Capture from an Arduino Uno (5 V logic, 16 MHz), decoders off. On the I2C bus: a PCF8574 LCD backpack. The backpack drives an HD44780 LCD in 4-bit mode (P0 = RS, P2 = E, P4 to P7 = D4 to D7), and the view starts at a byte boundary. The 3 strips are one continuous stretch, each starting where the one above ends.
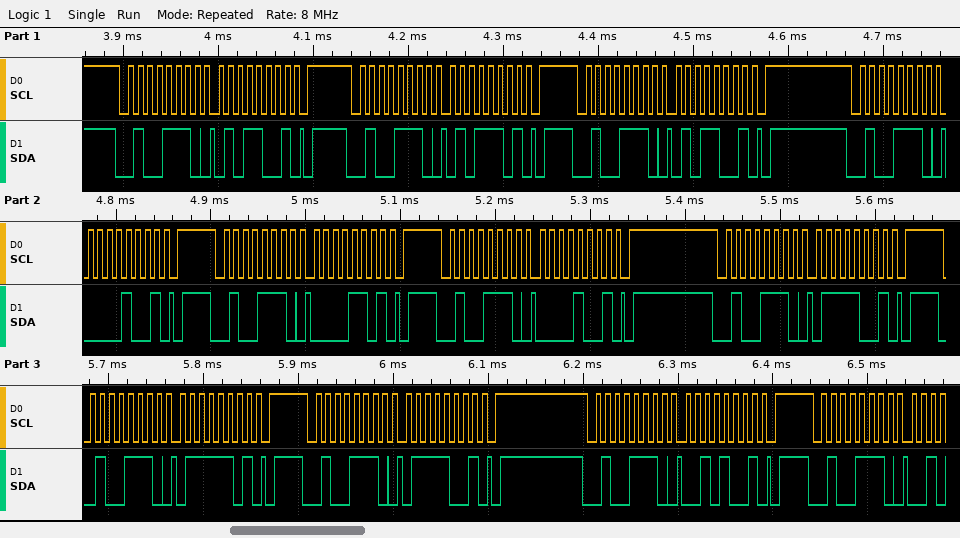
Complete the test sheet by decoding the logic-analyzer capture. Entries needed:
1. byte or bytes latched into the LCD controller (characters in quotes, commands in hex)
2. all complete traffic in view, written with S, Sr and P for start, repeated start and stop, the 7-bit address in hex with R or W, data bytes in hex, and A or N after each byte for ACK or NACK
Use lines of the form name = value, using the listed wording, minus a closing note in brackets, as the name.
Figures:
byte or bytes latched into the LCD controller = 'P'
all complete traffic in view, written with S, Sr and P for start, repeated start and stop, the 7-bit address in hex with R or W, data bytes in hex, and A or N after each byte for ACK or NACK = S 27W A 59 A P S 27W A 5D A P S 27W A 59 A P S 27W A 09 A P S 27W A 0D A P S 27W A 09 A P S 27W A 79 A P S 27W A 7D A P S 27W A 79 A P S 27W A 29 A P S 27W A
